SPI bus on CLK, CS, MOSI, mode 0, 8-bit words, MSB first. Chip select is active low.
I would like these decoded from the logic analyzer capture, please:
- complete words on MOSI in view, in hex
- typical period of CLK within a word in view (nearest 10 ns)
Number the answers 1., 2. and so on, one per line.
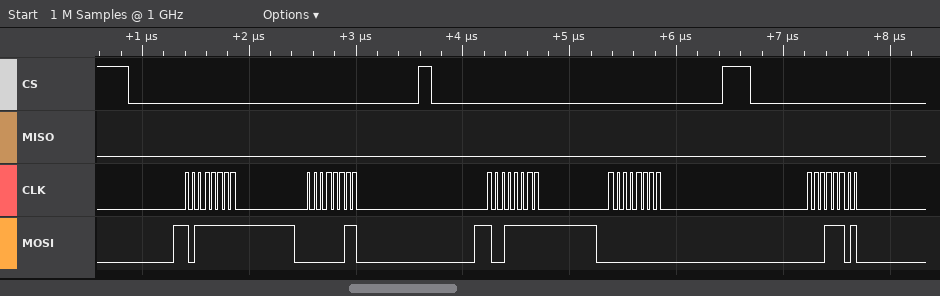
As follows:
1. BF, 03, 9F, 00, 1D
2. 60 ns
